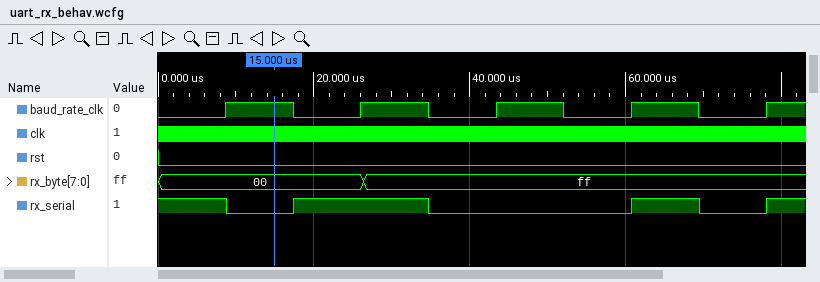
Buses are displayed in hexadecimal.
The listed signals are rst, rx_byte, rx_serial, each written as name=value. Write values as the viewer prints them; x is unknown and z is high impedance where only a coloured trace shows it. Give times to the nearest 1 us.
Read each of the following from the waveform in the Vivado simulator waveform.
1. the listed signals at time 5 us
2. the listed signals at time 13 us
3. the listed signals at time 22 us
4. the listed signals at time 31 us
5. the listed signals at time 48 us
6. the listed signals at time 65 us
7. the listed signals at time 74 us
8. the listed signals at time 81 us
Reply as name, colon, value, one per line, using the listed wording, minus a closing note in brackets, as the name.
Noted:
the listed signals at time 5 us: rst=0, rx_byte=00, rx_serial=1
the listed signals at time 13 us: rst=0, rx_byte=00, rx_serial=0
the listed signals at time 22 us: rst=0, rx_byte=00, rx_serial=1
the listed signals at time 31 us: rst=0, rx_byte=ff, rx_serial=1
the listed signals at time 48 us: rst=0, rx_byte=ff, rx_serial=0
the listed signals at time 65 us: rst=0, rx_byte=ff, rx_serial=1
the listed signals at time 74 us: rst=0, rx_byte=ff, rx_serial=0
the listed signals at time 81 us: rst=0, rx_byte=ff, rx_serial=1
